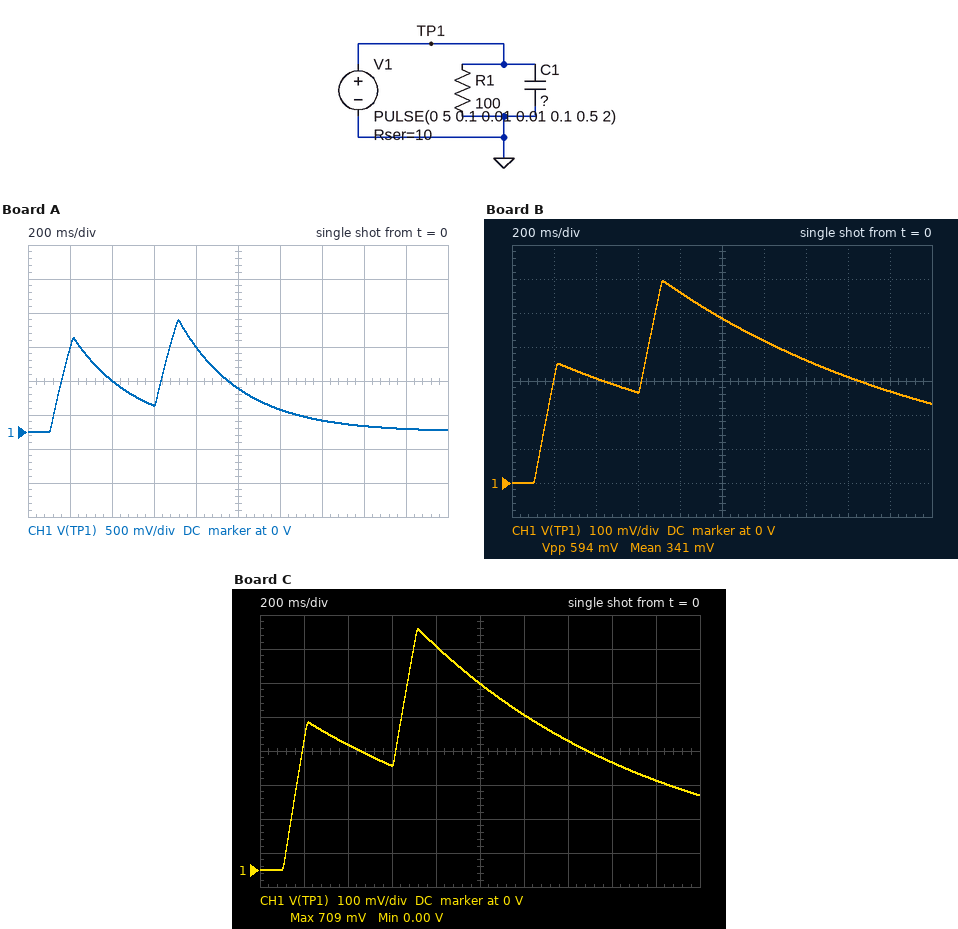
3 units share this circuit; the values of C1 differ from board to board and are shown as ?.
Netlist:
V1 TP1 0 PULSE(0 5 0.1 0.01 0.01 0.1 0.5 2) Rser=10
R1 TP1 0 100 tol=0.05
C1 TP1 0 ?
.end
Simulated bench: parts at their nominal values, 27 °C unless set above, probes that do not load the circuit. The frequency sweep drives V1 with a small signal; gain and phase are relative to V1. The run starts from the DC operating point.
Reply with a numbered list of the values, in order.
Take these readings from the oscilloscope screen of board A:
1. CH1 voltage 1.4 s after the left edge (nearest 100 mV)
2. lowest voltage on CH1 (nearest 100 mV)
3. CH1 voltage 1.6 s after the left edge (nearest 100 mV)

1. 200 mV
2. 0 V
3. 100 mV
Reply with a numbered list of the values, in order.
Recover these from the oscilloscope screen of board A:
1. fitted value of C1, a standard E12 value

1. 33 mF
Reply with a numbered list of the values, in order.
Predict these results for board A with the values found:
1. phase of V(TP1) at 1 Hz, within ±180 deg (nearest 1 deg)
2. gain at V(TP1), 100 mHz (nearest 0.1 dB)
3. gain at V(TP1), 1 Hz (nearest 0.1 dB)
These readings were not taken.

1. -62 deg
2. -1.0 dB
3. -7.4 dB
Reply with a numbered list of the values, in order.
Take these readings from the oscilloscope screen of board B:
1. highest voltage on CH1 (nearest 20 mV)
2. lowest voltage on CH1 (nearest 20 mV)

1. 600 mV
2. 0 V
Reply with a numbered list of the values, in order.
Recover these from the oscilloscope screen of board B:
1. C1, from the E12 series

1. 150 mF
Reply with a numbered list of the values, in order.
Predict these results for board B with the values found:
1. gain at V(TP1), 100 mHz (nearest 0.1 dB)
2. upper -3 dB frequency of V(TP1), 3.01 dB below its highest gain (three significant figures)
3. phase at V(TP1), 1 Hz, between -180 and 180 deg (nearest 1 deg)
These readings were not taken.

1. -3.2 dB
2. 117 mHz
3. -83 deg
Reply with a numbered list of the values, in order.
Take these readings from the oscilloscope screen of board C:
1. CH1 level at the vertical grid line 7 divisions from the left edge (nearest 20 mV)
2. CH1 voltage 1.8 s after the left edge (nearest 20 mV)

1. 380 mV
2. 260 mV
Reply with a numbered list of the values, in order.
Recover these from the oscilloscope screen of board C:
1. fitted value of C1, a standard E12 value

1. 120 mF
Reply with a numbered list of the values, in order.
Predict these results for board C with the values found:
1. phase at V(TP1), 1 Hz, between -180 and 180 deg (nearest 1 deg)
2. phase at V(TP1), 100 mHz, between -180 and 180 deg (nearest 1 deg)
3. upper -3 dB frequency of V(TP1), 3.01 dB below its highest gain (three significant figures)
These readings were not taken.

1. -82 deg
2. -34 deg
3. 146 mHz
